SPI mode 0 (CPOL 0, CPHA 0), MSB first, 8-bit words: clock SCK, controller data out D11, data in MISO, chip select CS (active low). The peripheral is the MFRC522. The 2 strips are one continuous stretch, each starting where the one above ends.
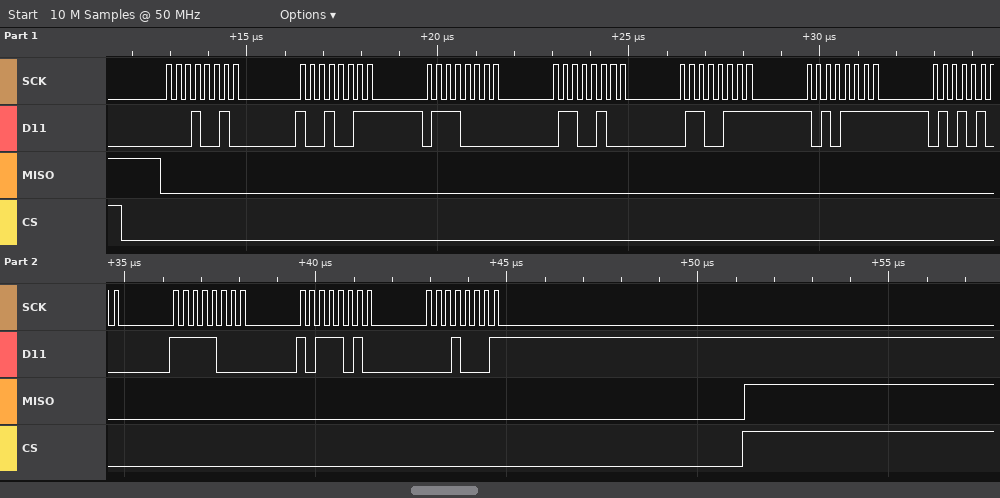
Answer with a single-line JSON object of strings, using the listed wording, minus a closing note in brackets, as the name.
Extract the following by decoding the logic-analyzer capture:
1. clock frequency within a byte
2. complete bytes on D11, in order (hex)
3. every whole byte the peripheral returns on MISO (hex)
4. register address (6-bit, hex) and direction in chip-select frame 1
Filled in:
{"clock frequency within a byte": "4 MHz", "complete bytes on D11, in order": "12 93 70 64 67 AF 54 F8 BA 11", "every whole byte the peripheral returns on MISO": "00 00 00 00 00 00 00 00 00 00", "register address (6-bit, hex) and direction in chip-select frame 1": "0x09 write"}
